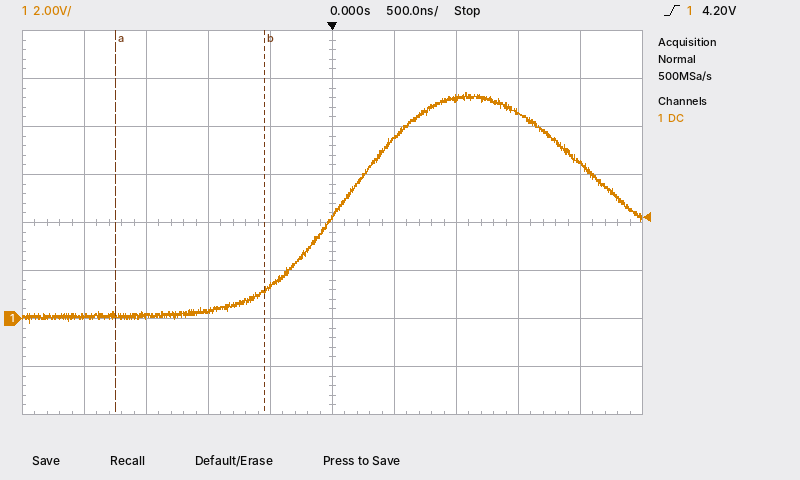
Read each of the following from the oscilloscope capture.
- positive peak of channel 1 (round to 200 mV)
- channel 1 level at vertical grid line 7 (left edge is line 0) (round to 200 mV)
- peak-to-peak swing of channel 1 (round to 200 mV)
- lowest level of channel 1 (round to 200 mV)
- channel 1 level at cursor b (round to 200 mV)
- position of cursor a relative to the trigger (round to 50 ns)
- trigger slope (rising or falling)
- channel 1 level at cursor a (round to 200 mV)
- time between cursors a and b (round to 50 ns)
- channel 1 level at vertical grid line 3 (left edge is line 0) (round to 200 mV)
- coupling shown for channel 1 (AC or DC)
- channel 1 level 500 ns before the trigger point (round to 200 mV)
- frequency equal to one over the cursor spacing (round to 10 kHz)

9.4 V
9.2 V
9.6 V
-200 mV
1.2 V
-1.75 µs
rising
200 mV
1.20 µs
400 mV
DC
1.4 V
830 kHz
